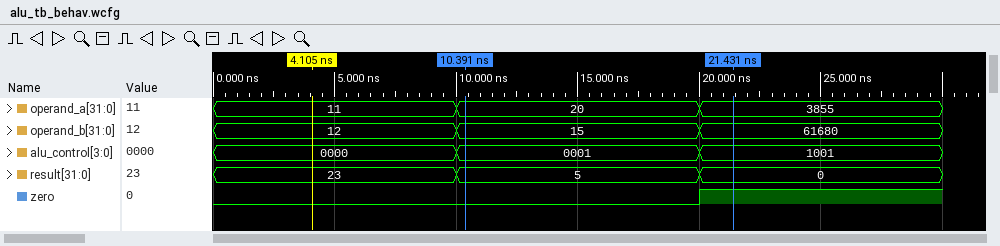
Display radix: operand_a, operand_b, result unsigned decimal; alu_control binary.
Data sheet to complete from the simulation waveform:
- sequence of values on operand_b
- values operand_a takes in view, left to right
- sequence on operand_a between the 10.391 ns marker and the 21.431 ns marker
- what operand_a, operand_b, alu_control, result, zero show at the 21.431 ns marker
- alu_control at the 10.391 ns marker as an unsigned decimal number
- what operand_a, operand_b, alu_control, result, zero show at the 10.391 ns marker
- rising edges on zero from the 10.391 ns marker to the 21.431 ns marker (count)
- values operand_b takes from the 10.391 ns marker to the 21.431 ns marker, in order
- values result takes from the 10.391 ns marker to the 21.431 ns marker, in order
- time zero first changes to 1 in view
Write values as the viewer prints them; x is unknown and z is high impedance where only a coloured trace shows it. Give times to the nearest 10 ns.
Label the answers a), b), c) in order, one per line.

a) 12, 15, 61680
b) 11, 20, 3855
c) 20, 3855
d) operand_a=3855, operand_b=61680, alu_control=1001, result=0, zero=1
e) 1
f) operand_a=20, operand_b=15, alu_control=0001, result=5, zero=0
g) 1
h) 15, 61680
i) 5, 0
j) 20 ns
